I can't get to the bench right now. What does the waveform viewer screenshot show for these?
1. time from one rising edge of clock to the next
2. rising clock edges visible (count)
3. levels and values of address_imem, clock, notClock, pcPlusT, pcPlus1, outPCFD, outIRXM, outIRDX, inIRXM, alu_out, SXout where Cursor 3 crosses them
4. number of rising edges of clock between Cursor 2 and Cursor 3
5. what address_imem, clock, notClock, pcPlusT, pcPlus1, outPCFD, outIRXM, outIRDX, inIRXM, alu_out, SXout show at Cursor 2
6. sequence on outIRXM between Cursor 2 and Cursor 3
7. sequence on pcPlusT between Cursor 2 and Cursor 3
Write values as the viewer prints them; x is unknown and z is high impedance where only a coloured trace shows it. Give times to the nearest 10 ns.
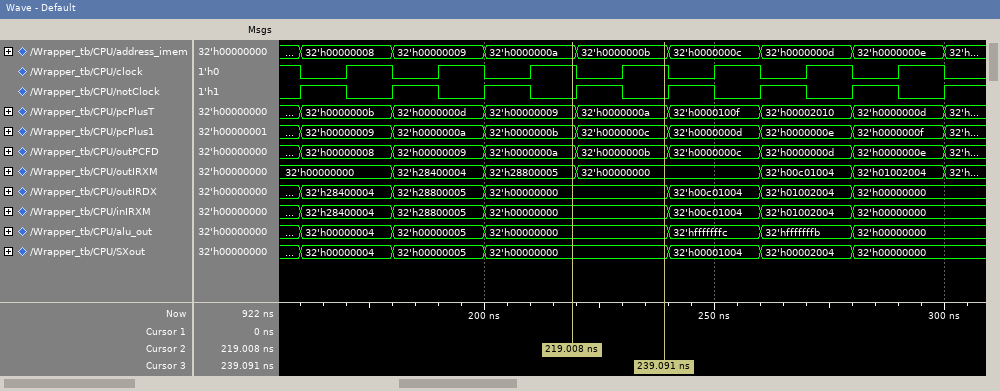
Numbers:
20 ns
7
address_imem=32'h0000000b, clock=1, notClock=0, pcPlusT=32'h0000000a, pcPlus1=32'h0000000c, outPCFD=32'h0000000b, outIRXM=32'h00000000, outIRDX=32'h00000000, inIRXM=32'h00000000, alu_out=32'h00000000, SXout=32'h00000000
1
address_imem=32'h0000000a, clock=1, notClock=0, pcPlusT=32'h00000009, pcPlus1=32'h0000000b, outPCFD=32'h0000000a, outIRXM=32'h28800005, outIRDX=32'h00000000, inIRXM=32'h00000000, alu_out=32'h00000000, SXout=32'h00000000
32'h28800005, 32'h00000000
32'h00000009, 32'h0000000a
